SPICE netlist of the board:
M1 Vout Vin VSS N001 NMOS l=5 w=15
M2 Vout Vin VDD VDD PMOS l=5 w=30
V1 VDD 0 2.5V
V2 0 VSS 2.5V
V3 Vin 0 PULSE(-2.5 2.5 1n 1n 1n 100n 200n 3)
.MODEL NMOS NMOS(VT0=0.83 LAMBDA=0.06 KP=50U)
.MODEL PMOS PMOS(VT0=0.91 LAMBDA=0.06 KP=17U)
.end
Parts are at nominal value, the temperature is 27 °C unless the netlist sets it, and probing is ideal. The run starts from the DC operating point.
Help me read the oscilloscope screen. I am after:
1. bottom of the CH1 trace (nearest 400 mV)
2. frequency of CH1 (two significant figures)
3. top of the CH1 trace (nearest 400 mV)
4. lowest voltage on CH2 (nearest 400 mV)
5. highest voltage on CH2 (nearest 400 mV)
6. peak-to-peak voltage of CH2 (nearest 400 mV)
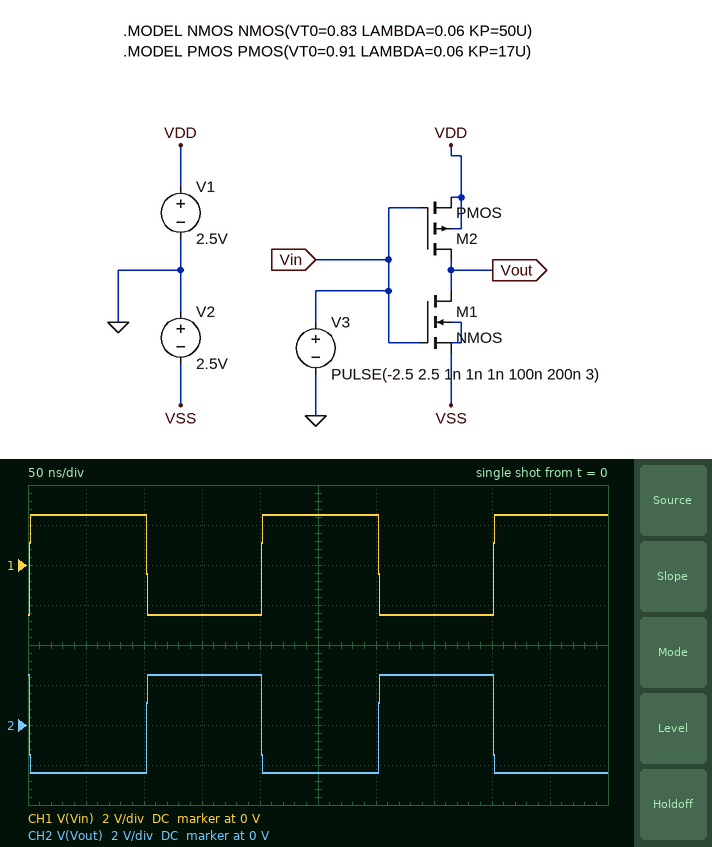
-2.4 V
5.0 MHz
2.4 V
-2.4 V
2.4 V
4.8 V
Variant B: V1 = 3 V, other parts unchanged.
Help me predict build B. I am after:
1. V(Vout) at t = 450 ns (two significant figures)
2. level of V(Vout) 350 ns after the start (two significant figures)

-2.3 V
3.0 V
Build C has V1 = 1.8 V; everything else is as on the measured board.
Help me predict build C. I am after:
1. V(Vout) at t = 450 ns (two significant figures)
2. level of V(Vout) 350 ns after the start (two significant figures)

-2.5 V
1.8 V
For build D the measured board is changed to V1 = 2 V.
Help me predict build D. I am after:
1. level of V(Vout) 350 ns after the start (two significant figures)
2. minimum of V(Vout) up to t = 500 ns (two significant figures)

2.0 V
-2.5 V
